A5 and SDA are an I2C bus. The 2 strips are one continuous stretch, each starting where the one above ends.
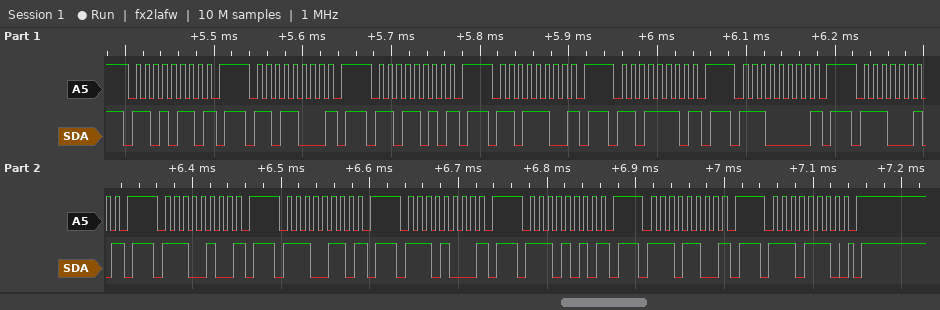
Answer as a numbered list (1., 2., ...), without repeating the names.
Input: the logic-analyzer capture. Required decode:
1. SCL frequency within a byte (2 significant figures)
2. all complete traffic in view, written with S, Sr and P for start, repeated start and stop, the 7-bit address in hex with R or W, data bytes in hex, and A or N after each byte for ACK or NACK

1. 100 kHz
2. S 6BW N P S 6CW N P S 6DW N P S 6EW N P S 6FW N P S 70W N P S 71W N P S 72W N P S 73W N P S 74W N P S 75W N P S 76W N P S 77W A P
